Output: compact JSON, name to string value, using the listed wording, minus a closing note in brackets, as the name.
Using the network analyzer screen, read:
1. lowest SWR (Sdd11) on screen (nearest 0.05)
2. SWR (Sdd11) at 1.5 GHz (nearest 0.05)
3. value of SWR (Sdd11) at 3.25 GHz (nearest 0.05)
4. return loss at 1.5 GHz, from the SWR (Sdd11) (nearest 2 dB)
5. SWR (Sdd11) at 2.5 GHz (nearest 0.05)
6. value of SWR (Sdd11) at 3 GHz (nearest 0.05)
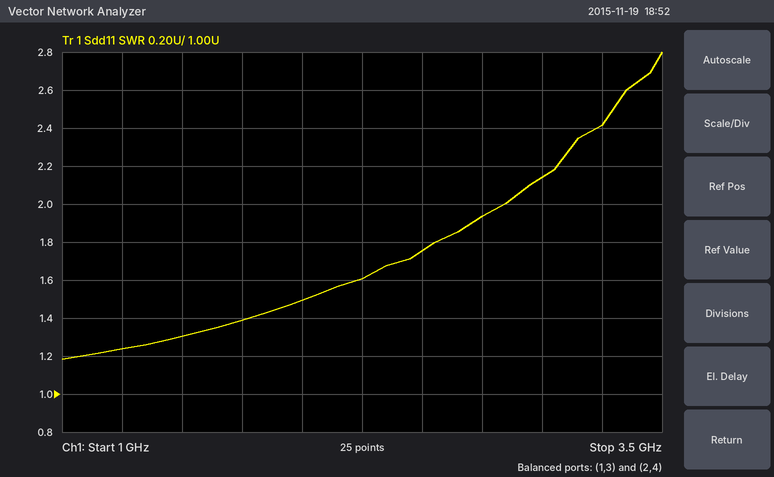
{"lowest SWR (Sdd11) on screen": "1.20", "SWR (Sdd11) at 1.5 GHz": "1.30", "value of SWR (Sdd11) at 3.25 GHz": "2.40", "return loss at 1.5 GHz, from the SWR (Sdd11)": "18 dB", "SWR (Sdd11) at 2.5 GHz": "1.75", "value of SWR (Sdd11) at 3 GHz": "2.15"}
